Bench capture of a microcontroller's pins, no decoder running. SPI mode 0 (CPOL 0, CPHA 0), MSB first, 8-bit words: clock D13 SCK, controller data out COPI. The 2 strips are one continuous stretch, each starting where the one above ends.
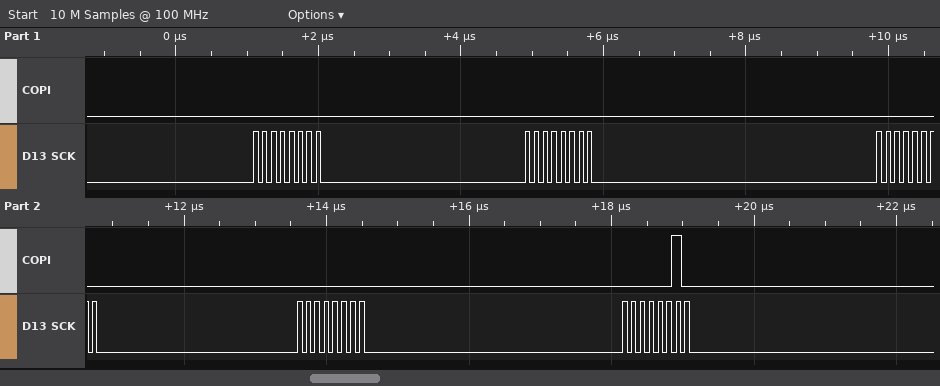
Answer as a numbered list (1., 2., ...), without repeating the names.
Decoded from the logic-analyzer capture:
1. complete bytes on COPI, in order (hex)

1. 00 00 00 00 02
